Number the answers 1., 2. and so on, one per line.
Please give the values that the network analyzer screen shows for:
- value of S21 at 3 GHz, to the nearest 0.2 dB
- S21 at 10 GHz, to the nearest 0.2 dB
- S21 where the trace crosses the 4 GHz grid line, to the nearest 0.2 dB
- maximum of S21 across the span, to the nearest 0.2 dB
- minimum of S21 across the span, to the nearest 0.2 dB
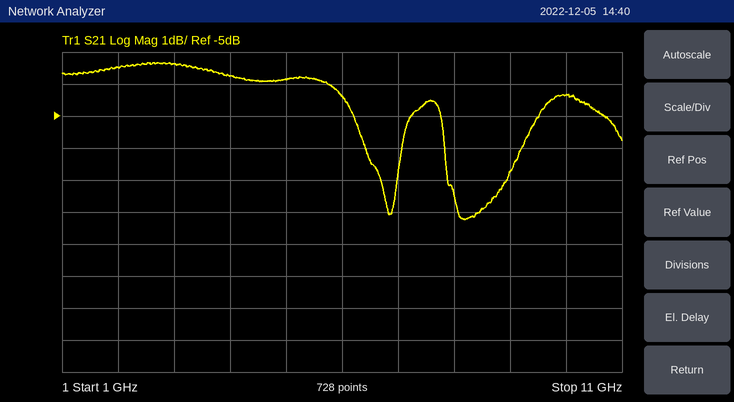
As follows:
1. -3.4 dB
2. -4.4 dB
3. -3.8 dB
4. -3.4 dB
5. -8.2 dB
